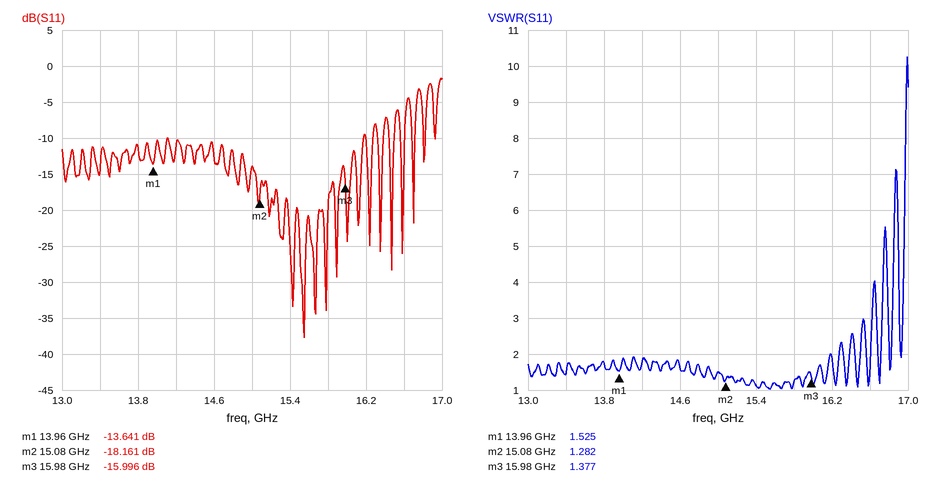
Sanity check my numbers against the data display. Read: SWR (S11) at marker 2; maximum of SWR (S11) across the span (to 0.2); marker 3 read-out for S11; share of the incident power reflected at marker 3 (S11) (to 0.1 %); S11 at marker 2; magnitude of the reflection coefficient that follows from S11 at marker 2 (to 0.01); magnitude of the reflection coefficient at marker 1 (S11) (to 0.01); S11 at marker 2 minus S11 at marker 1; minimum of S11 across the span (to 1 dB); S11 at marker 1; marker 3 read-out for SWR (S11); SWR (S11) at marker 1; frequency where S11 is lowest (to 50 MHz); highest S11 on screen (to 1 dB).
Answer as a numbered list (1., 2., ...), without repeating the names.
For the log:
1. 1.282
2. 10.2
3. -15.996 dB
4. 2.5 %
5. -18.161 dB
6. 0.12
7. 0.21
8. -4.520 dB
9. -38 dB
10. -13.641 dB
11. 1.377
12. 1.525
13. 15.55 GHz
14. -2 dB
